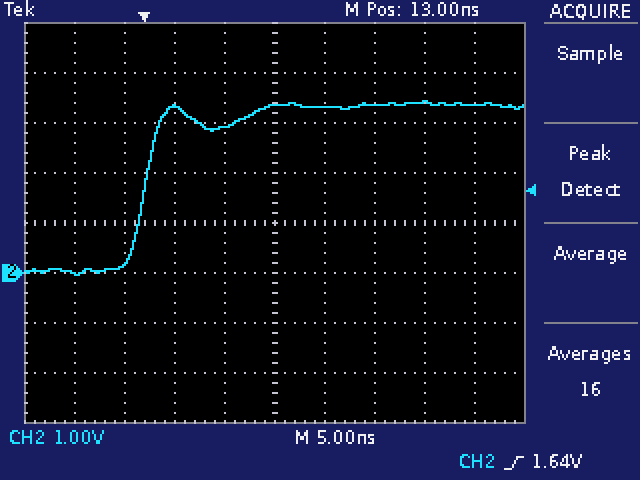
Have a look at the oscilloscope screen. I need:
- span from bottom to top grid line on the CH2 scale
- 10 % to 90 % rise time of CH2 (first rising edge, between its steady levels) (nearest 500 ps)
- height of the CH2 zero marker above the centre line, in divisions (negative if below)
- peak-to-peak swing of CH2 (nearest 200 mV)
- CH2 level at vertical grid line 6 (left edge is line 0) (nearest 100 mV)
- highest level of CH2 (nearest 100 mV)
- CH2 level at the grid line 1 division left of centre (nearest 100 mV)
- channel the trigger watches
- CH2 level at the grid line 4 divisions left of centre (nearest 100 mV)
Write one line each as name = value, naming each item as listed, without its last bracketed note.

span from bottom to top grid line on the CH2 scale = 8 V
10 % to 90 % rise time of CH2 (first rising edge, between its steady levels) = 3.0 ns
height of the CH2 zero marker above the centre line, in divisions = -1.0 div
peak-to-peak swing of CH2 = 3.4 V
CH2 level at vertical grid line 6 (left edge is line 0) = 3.3 V
highest level of CH2 = 3.4 V
CH2 level at the grid line 1 division left of centre = 2.9 V
channel the trigger watches = CH2
CH2 level at the grid line 4 divisions left of centre = 0.0 V
